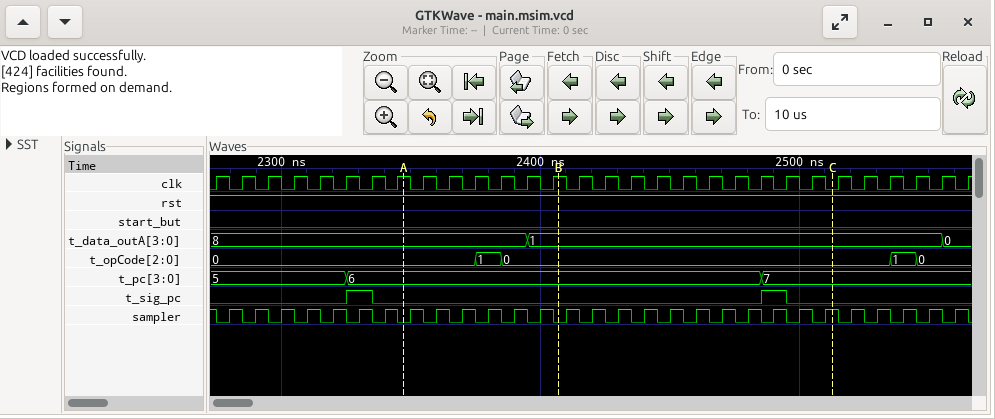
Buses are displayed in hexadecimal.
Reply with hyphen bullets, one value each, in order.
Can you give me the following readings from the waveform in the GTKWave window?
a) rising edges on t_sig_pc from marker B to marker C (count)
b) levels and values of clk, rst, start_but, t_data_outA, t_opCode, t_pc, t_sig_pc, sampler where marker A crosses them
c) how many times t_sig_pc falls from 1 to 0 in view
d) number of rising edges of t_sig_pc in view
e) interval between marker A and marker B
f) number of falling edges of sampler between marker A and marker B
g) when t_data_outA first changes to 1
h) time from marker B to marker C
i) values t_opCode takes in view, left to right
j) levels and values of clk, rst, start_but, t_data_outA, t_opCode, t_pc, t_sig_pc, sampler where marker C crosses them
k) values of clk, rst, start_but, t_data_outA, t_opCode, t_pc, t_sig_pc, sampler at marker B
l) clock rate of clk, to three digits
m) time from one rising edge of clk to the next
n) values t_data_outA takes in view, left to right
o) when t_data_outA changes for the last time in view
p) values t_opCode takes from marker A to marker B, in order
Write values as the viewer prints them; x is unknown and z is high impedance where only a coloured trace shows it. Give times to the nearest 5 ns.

- 1
- clk=1, rst=1, start_but=0, t_data_outA=8, t_opCode=0, t_pc=6, t_sig_pc=0, sampler=0
- 2
- 2
- 60 ns
- 6
- 2395 ns
- 105 ns
- 0, 1, 0, 1, 0
- clk=0, rst=1, start_but=0, t_data_outA=1, t_opCode=0, t_pc=7, t_sig_pc=0, sampler=1
- clk=1, rst=1, start_but=0, t_data_outA=1, t_opCode=0, t_pc=6, t_sig_pc=0, sampler=0
- 100 MHz
- 10 ns
- 8, 1, 0
- 2555 ns
- 0, 1, 0
